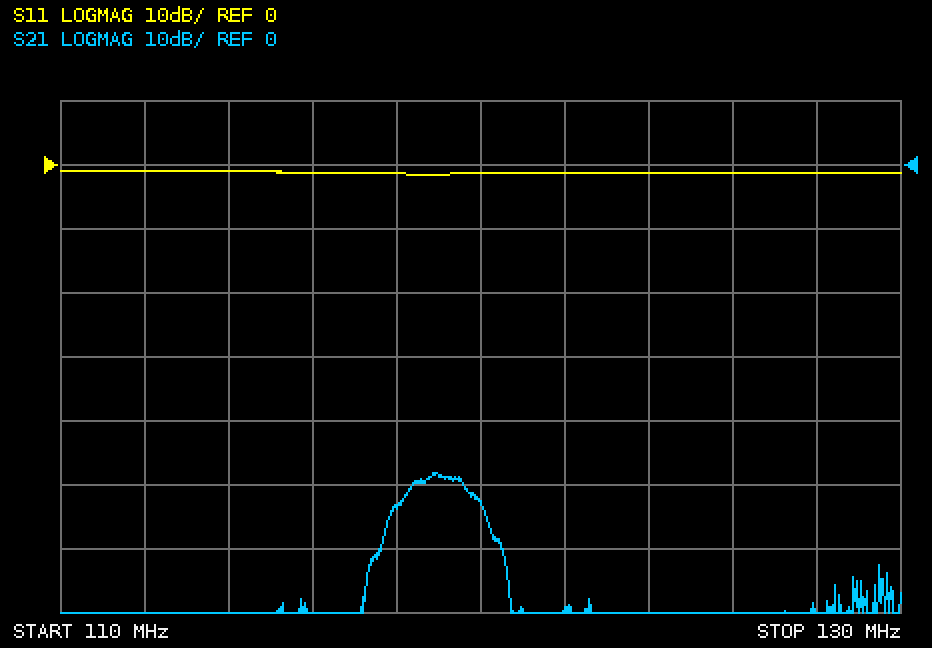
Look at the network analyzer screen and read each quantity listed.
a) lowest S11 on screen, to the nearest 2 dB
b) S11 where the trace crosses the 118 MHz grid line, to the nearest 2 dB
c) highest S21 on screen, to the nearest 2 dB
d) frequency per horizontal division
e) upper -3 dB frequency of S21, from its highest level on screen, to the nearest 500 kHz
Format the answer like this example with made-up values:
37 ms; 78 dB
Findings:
-2 dB; -2 dB; -48 dB; 2 MHz; 119.5 MHz
